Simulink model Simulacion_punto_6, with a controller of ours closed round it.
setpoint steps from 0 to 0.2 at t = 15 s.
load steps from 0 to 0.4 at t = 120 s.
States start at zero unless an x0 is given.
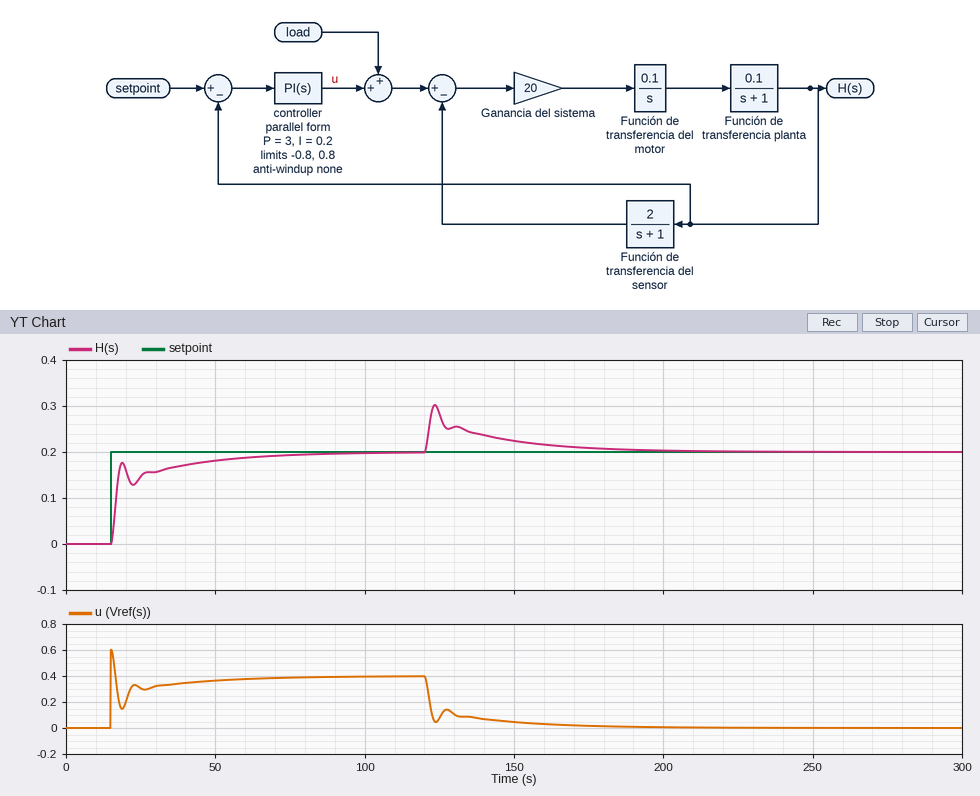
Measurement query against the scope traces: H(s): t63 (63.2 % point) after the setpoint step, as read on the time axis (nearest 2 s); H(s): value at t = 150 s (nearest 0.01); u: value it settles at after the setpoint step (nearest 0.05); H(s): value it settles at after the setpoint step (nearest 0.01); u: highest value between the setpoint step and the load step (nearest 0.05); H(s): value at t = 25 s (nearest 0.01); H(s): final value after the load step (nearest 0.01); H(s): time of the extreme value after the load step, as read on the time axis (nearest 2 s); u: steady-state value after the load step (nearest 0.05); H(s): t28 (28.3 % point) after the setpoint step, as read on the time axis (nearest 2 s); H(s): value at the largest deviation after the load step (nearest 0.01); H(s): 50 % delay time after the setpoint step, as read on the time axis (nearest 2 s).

18 s
0.22
0.40
0.20
0.60
0.15
0.20
124 s
0.00
16 s
0.30
16 s
